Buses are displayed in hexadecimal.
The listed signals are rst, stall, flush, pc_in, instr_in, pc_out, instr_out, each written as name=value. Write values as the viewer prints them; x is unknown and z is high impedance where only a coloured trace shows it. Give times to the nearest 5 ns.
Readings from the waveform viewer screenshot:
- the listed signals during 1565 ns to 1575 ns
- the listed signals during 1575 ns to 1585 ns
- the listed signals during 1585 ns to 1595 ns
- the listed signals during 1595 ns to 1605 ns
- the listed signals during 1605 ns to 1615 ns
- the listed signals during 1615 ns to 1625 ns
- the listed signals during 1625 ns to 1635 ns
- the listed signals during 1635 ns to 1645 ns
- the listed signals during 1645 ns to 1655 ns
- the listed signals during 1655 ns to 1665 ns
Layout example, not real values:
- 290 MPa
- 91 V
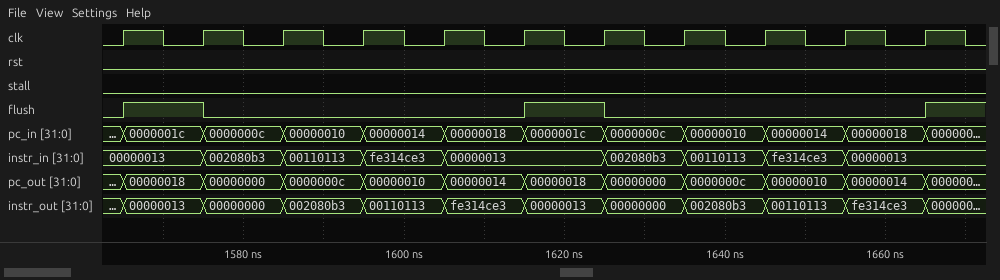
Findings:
- rst=0, stall=0, flush=1, pc_in=0000001c, instr_in=00000013, pc_out=00000018, instr_out=00000013
- rst=0, stall=0, flush=0, pc_in=0000000c, instr_in=002080b3, pc_out=00000000, instr_out=00000000
- rst=0, stall=0, flush=0, pc_in=00000010, instr_in=00110113, pc_out=0000000c, instr_out=002080b3
- rst=0, stall=0, flush=0, pc_in=00000014, instr_in=fe314ce3, pc_out=00000010, instr_out=00110113
- rst=0, stall=0, flush=0, pc_in=00000018, instr_in=00000013, pc_out=00000014, instr_out=fe314ce3
- rst=0, stall=0, flush=1, pc_in=0000001c, instr_in=00000013, pc_out=00000018, instr_out=00000013
- rst=0, stall=0, flush=0, pc_in=0000000c, instr_in=002080b3, pc_out=00000000, instr_out=00000000
- rst=0, stall=0, flush=0, pc_in=00000010, instr_in=00110113, pc_out=0000000c, instr_out=002080b3
- rst=0, stall=0, flush=0, pc_in=00000014, instr_in=fe314ce3, pc_out=00000010, instr_out=00110113
- rst=0, stall=0, flush=0, pc_in=00000018, instr_in=00000013, pc_out=00000014, instr_out=fe314ce3
